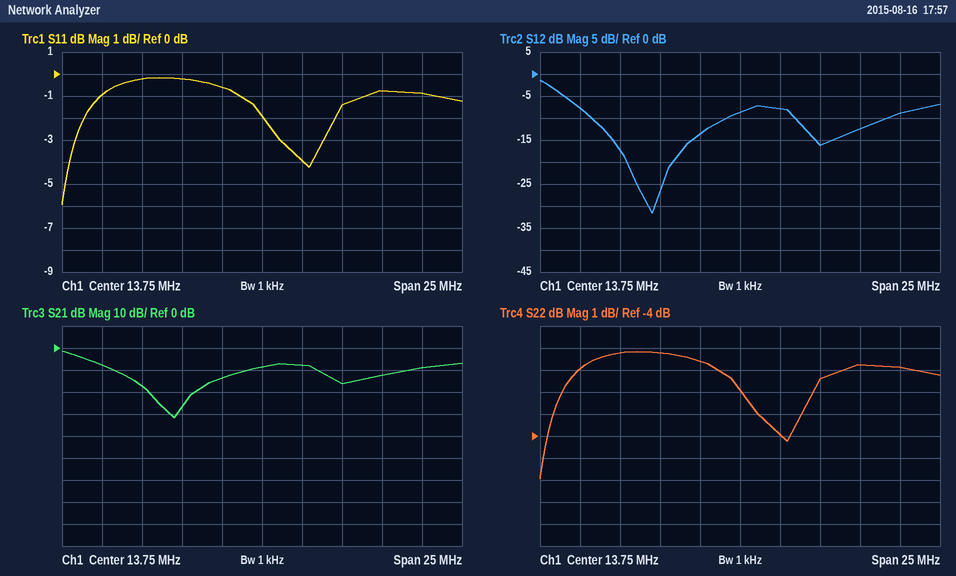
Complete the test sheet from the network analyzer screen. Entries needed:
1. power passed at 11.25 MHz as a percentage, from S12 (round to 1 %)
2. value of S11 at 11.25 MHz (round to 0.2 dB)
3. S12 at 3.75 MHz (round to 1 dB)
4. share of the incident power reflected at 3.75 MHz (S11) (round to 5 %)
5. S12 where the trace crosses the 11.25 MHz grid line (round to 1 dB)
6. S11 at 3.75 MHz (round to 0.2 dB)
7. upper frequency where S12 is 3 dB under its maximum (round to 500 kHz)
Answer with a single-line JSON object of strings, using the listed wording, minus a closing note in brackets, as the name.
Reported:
{"power passed at 11.25 MHz as a percentage, from S12": "4 %", "value of S11 at 11.25 MHz": "-0.6 dB", "S12 at 3.75 MHz": "-8 dB", "share of the incident power reflected at 3.75 MHz (S11)": "80 %", "S12 where the trace crosses the 11.25 MHz grid line": "-14 dB", "S11 at 3.75 MHz": "-1.0 dB", "upper frequency where S12 is 3 dB under its maximum": "2.5 MHz"}
